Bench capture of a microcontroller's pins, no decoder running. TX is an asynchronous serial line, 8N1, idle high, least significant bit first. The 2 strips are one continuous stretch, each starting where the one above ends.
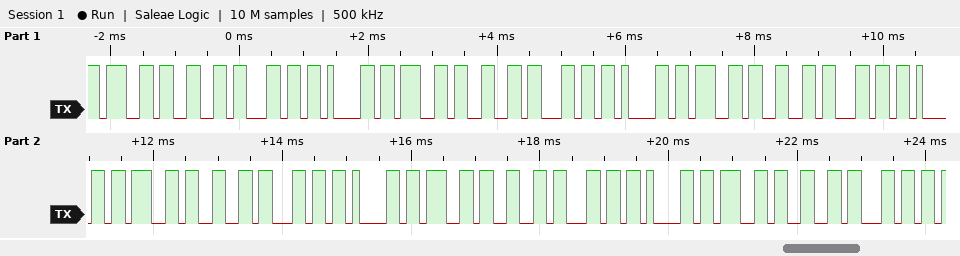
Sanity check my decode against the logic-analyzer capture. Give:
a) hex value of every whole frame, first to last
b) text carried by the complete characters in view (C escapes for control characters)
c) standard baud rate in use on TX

67 66 6C 61 67 66 6C 61 67 66 6C 61 67 66 6C 61 67 66 6C 61 67 66 6C
"gflagflagflagflagflagfl"
9600 baud
